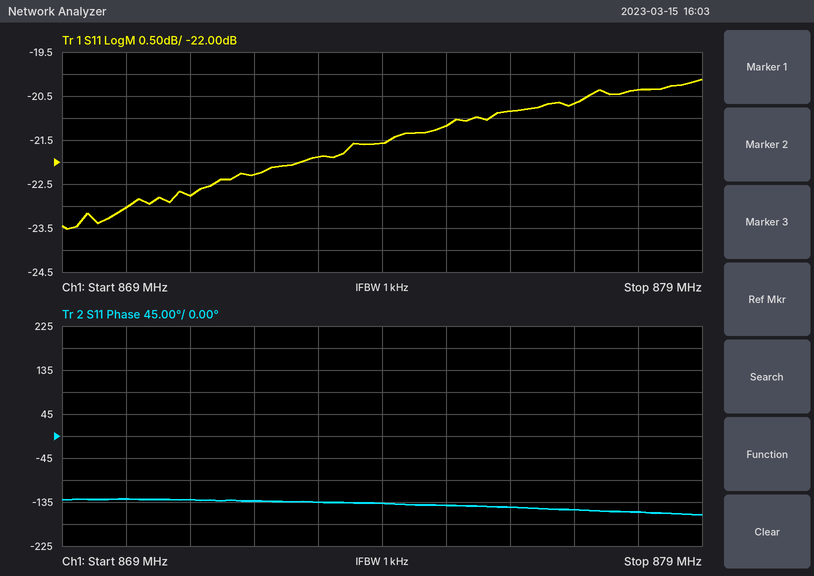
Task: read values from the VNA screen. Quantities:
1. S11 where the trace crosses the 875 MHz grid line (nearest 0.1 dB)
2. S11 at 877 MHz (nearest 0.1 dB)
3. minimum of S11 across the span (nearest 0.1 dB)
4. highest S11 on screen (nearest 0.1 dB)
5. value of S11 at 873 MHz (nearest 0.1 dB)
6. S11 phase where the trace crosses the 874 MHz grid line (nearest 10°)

-21.2 dB
-20.7 dB
-23.5 dB
-20.1 dB
-21.9 dB
-140°
